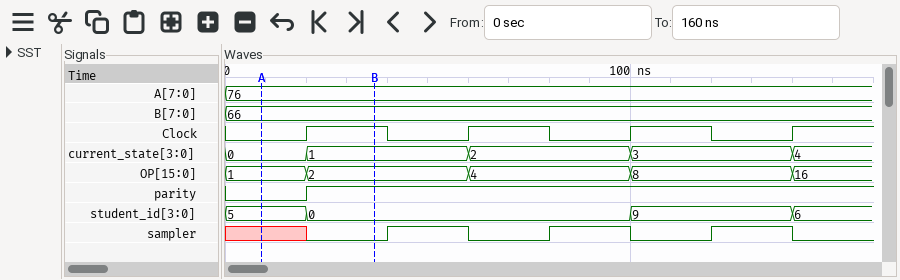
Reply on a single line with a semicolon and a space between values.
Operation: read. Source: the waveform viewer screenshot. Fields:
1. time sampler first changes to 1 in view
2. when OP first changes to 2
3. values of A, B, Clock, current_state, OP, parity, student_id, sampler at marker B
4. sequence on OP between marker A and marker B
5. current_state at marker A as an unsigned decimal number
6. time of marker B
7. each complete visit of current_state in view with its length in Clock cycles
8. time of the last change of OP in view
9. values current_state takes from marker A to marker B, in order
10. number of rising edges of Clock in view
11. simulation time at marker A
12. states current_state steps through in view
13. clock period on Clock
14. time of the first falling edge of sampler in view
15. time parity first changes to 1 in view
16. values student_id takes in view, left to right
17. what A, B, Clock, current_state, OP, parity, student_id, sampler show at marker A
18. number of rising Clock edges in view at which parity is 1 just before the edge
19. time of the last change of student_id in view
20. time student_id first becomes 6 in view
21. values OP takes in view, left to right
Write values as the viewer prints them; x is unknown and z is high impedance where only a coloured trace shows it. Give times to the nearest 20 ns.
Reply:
40 ns; 20 ns; A=76, B=66, Clock=1, current_state=1, OP=2, parity=1, student_id=0, sampler=0; 1, 2; 0; 40 ns; 1: 1, 2: 1, 3: 1; 140 ns; 0, 1; 4; 0 ns; 0, 1, 2, 3, 4; 40 ns; 60 ns; 20 ns; 5, 0, 9, 6; A=76, B=66, Clock=0, current_state=0, OP=1, parity=0, student_id=5, sampler=x; 3; 140 ns; 140 ns; 1, 2, 4, 8, 16
